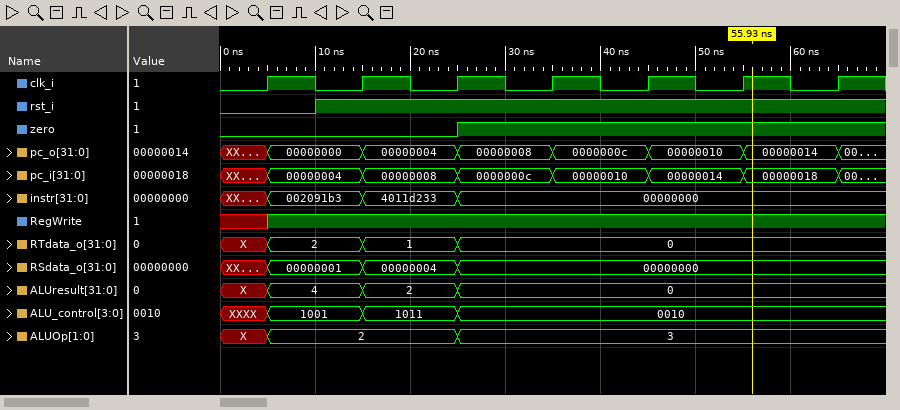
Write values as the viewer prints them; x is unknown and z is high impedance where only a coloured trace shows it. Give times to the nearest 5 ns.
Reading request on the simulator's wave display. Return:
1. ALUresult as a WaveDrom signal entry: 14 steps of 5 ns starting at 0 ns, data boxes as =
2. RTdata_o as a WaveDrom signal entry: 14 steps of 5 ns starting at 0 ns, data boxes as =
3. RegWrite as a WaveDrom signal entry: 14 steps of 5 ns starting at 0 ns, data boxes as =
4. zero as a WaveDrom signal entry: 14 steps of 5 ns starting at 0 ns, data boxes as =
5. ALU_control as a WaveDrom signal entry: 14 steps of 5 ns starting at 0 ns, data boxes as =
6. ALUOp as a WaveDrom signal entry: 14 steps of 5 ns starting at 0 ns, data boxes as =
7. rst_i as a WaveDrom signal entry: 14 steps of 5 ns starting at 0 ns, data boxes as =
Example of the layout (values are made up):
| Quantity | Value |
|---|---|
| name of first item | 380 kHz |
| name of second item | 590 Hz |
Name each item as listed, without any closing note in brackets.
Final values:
| Quantity | Value |
|---|---|
| ALUresult as a WaveDrom signal entry: 14 steps of 5 ns starting at 0 ns, data boxes as = | {name: 'ALUresult', wave: 'x=.=.=........', data: '4 2 0'} |
| RTdata_o as a WaveDrom signal entry: 14 steps of 5 ns starting at 0 ns, data boxes as = | {name: 'RTdata_o', wave: 'x=.=.=........', data: '2 1 0'} |
| RegWrite as a WaveDrom signal entry: 14 steps of 5 ns starting at 0 ns, data boxes as = | {name: 'RegWrite', wave: 'x1............'} |
| zero as a WaveDrom signal entry: 14 steps of 5 ns starting at 0 ns, data boxes as = | {name: 'zero', wave: '0....1........'} |
| ALU_control as a WaveDrom signal entry: 14 steps of 5 ns starting at 0 ns, data boxes as = | {name: 'ALU_control', wave: 'x=.=.=........', data: '1001 1011 0010'} |
| ALUOp as a WaveDrom signal entry: 14 steps of 5 ns starting at 0 ns, data boxes as = | {name: 'ALUOp', wave: 'x=...=........', data: '2 3'} |
| rst_i as a WaveDrom signal entry: 14 steps of 5 ns starting at 0 ns, data boxes as = | {name: 'rst_i', wave: '0.1...........'} |
